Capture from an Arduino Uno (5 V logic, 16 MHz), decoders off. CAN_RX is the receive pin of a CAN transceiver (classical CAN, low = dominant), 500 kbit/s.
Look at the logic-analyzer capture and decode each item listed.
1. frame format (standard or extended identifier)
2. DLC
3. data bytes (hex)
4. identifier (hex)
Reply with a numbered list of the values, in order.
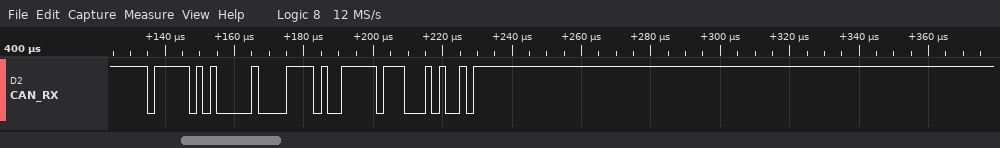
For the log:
1. standard
2. 1
3. E9
4. 0x7E8
